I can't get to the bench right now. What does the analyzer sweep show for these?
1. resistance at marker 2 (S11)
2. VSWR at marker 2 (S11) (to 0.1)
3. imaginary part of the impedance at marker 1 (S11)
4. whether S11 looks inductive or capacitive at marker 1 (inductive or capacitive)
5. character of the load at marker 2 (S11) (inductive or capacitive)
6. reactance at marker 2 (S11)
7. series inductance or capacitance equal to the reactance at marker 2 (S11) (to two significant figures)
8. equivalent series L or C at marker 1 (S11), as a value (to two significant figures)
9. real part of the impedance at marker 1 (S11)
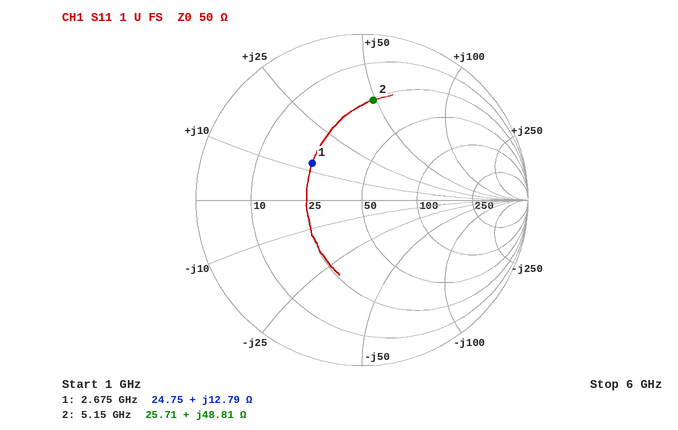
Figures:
25.71 Ω
4.1
+12.79 Ω
inductive
inductive
+48.81 Ω
1.5 nH
760 pH
24.75 Ω
